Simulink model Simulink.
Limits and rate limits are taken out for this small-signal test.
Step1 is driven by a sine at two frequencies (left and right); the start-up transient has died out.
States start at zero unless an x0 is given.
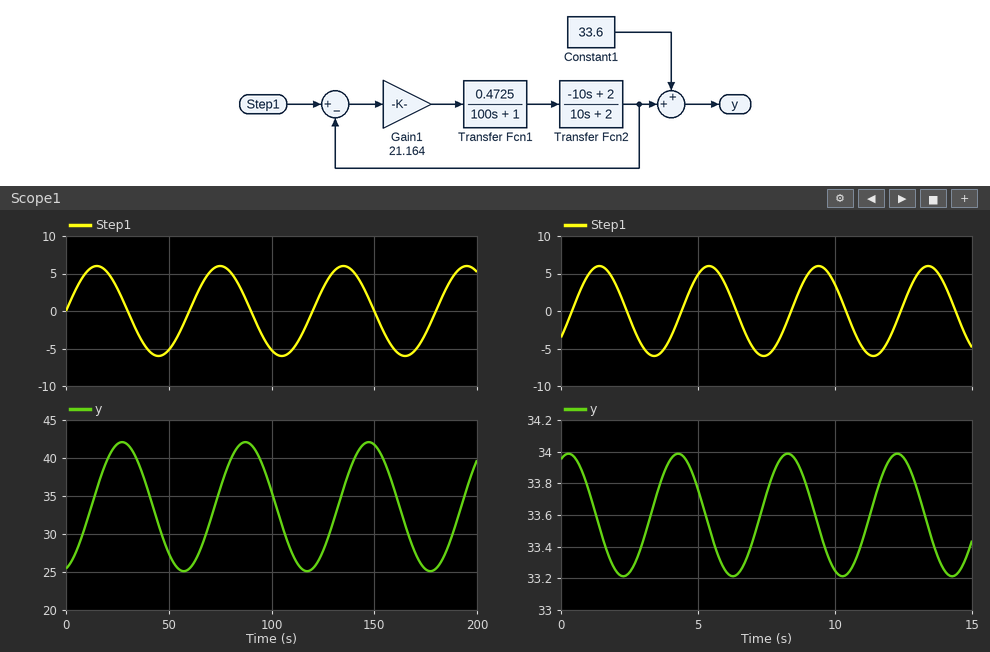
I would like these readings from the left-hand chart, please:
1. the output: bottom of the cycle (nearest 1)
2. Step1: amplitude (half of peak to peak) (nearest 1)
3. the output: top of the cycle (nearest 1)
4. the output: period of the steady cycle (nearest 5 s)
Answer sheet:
25
6
42
60 s
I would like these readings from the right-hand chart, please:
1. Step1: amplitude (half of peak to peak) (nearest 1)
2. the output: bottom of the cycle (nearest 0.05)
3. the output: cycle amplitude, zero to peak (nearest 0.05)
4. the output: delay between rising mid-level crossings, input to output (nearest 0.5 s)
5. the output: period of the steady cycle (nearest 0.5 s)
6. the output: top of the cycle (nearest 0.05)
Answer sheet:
6
33.20
0.40
3.0 s
4.0 s
34.00
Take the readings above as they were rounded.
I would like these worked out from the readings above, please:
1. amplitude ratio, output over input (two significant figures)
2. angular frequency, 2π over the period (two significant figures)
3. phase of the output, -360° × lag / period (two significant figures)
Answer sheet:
0.067
1.6 rad/s
-270°
